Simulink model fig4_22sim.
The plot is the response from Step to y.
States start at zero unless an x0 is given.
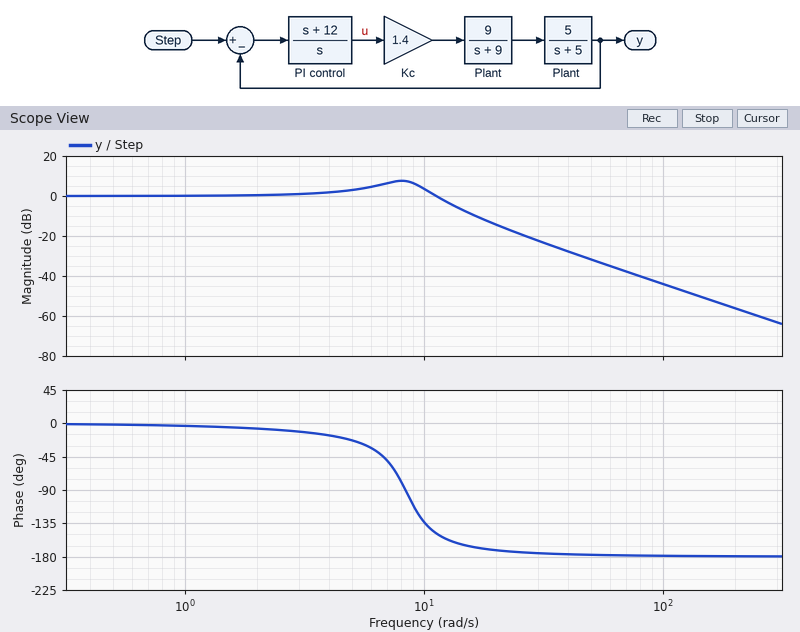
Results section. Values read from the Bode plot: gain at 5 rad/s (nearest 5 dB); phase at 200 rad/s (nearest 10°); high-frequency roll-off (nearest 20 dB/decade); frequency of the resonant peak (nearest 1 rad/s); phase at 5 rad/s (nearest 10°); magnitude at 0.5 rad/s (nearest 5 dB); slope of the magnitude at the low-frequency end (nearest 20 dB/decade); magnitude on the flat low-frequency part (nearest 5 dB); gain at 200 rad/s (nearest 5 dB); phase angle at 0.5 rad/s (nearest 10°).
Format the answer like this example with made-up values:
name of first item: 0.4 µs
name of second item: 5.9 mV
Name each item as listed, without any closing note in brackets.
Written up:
gain at 5 rad/s: 5 dB
phase at 200 rad/s: -180°
high-frequency roll-off: -40 dB/decade
frequency of the resonant peak: 8 rad/s
phase at 5 rad/s: -20°
magnitude at 0.5 rad/s: 0 dB
slope of the magnitude at the low-frequency end: 0 dB/decade
magnitude on the flat low-frequency part: 0 dB
gain at 200 rad/s: -55 dB
phase angle at 0.5 rad/s: 0°
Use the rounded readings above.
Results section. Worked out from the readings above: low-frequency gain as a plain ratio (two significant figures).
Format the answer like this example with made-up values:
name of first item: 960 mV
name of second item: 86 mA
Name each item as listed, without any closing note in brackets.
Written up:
low-frequency gain as a plain ratio: 1.0
